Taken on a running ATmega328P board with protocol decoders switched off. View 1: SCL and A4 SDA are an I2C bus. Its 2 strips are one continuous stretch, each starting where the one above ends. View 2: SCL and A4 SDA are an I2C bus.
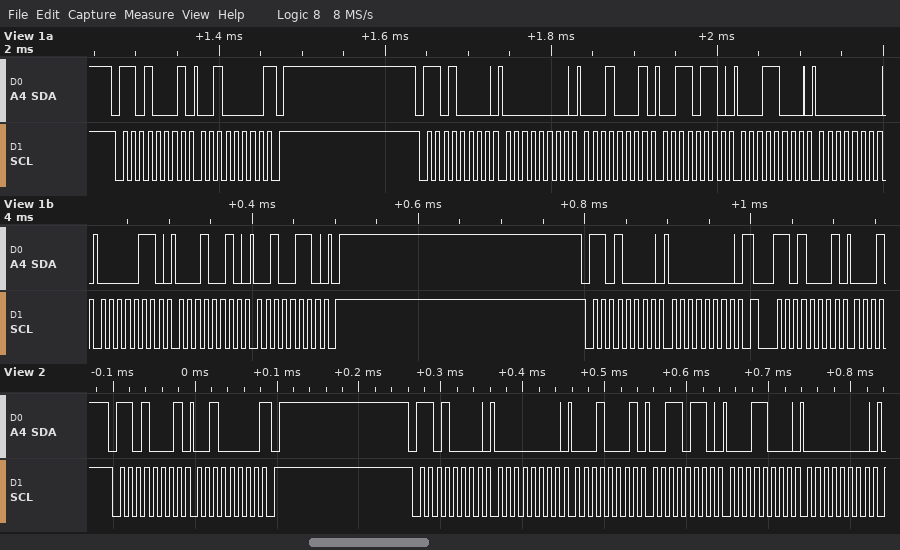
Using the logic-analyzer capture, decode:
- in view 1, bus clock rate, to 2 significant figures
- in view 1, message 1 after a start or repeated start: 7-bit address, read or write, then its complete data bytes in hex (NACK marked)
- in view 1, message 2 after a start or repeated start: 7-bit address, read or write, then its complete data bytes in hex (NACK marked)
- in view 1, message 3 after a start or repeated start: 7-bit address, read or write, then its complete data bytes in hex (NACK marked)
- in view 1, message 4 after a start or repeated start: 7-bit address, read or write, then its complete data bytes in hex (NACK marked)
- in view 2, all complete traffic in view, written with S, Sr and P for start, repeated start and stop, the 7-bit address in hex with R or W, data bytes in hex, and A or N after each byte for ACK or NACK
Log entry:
100 kHz
0x68 read: 20 NACK
0x68 write: 00 11 36 18 00 06 12 26
0x68 write: 00
0x68 read
S 68R A 20 N P S 68W A 00 A 11 A 36 A 18 A 00 A
